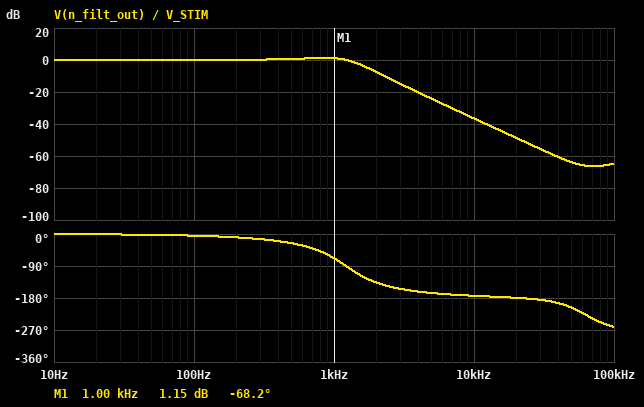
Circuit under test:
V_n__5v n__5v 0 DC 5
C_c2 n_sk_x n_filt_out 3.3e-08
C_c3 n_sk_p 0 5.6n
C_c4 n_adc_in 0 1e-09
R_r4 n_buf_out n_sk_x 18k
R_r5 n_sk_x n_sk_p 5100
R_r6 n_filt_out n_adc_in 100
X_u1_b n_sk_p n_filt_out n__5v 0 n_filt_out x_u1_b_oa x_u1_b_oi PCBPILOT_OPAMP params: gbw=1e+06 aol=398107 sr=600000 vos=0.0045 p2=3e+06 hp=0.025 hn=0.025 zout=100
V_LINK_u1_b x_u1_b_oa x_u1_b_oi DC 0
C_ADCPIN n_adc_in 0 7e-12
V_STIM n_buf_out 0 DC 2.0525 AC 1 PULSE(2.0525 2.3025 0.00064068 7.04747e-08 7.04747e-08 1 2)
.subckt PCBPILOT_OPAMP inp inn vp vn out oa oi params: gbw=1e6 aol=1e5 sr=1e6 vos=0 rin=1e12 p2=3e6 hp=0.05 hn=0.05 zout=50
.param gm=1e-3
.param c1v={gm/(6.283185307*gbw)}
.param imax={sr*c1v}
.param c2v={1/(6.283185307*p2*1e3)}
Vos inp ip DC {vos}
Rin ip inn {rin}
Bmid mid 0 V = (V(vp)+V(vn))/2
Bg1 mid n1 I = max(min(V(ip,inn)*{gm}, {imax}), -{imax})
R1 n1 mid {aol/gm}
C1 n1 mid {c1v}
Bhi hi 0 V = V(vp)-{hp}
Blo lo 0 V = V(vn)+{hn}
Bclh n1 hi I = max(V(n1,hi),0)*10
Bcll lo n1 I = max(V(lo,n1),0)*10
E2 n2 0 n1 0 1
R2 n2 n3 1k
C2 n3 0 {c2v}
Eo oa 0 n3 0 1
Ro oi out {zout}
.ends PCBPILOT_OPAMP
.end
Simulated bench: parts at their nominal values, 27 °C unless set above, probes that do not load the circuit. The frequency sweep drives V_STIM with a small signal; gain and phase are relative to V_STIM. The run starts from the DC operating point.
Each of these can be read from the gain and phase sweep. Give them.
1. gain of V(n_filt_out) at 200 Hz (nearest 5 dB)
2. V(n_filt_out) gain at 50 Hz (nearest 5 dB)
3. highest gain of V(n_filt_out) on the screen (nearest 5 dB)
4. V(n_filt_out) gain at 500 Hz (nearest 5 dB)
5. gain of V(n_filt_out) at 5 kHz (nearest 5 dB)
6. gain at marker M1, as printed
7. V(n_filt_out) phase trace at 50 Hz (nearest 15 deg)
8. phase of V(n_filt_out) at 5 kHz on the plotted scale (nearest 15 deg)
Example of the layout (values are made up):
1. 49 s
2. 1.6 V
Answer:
1. 0 dB
2. 0 dB
3. 0 dB
4. 0 dB
5. -25 dB
6. 1.15 dB
7. 0 deg
8. -165 deg
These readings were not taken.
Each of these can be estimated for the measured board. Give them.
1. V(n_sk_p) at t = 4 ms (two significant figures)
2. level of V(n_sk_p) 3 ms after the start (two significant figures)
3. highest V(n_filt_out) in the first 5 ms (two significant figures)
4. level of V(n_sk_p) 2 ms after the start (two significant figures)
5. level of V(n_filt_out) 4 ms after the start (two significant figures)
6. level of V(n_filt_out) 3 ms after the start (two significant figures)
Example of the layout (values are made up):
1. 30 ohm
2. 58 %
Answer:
1. 2.3 V
2. 2.3 V
3. 2.3 V
4. 2.3 V
5. 2.3 V
6. 2.3 V
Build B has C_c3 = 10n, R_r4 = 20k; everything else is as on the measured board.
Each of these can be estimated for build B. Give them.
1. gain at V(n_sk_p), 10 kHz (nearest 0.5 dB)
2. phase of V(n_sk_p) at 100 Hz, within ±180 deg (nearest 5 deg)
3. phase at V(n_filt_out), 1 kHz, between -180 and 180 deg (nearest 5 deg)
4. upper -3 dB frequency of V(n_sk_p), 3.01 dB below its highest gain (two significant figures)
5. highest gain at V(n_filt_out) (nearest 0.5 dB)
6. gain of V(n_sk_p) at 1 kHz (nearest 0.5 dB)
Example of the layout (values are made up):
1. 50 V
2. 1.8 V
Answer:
1. -42.5 dB
2. -10 deg
3. -100 deg
4. 890 Hz
5. 0 dB
6. -4.0 dB
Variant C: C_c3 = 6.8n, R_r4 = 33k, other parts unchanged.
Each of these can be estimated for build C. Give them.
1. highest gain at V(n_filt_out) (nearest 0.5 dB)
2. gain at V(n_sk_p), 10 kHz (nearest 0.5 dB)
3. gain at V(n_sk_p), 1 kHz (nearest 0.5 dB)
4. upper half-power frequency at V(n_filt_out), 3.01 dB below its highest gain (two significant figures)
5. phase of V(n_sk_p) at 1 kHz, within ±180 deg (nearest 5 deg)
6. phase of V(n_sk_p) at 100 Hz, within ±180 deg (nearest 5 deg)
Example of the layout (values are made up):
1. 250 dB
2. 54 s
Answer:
1. 0 dB
2. -43.5 dB
3. -4.5 dB
4. 860 Hz
5. -105 deg
6. -10 deg
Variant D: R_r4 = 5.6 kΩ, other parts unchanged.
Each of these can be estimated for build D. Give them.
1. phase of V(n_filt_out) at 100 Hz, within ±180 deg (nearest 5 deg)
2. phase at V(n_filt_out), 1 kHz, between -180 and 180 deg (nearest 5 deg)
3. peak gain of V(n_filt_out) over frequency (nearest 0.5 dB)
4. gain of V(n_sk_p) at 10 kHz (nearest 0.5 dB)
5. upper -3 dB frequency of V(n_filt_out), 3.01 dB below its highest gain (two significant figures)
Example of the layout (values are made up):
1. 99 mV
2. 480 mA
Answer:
1. 0 deg
2. -25 deg
3. 2.5 dB
4. -26.0 dB
5. 2.6 kHz
